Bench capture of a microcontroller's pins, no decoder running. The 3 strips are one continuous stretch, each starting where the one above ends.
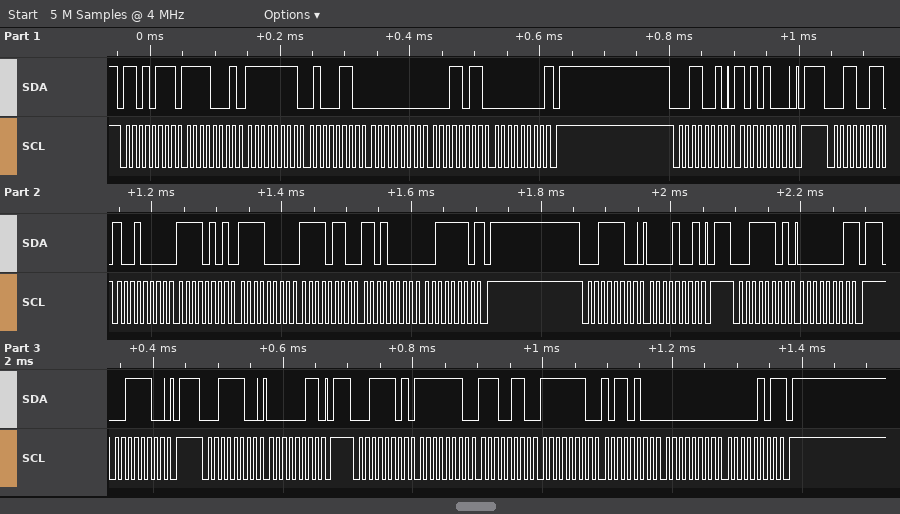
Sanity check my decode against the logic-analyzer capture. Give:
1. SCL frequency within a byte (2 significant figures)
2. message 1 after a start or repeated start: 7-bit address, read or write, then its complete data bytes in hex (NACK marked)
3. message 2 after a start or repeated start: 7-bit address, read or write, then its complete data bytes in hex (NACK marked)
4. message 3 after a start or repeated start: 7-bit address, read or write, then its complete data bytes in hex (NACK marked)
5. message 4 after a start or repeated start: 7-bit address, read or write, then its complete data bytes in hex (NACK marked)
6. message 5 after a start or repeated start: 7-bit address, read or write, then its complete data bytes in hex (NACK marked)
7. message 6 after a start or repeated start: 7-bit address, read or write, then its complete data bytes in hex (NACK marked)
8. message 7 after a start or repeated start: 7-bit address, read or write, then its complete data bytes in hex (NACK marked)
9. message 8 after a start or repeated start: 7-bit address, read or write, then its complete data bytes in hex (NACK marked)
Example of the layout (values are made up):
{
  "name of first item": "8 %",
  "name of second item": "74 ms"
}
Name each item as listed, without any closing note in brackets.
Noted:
{
  "SCL frequency within a byte": "100 kHz",
  "message 1 after a start or repeated start: 7-bit address, read or write, then its complete data bytes in hex": "0x6B read: F1 FF 46 00 1B 00 NACK",
  "message 2 after a start or repeated start: 7-bit address, read or write, then its complete data bytes in hex": "0x19 write: A8",
  "message 3 after a start or repeated start: 7-bit address, read or write, then its complete data bytes in hex": "0x19 read: 90 F5 F0 F6 D0 3E NACK",
  "message 4 after a start or repeated start: 7-bit address, read or write, then its complete data bytes in hex": "0x1E write: 09",
  "message 5 after a start or repeated start: 7-bit address, read or write, then its complete data bytes in hex": "0x1E read: 01 NACK",
  "message 6 after a start or repeated start: 7-bit address, read or write, then its complete data bytes in hex": "0x1E write",
  "message 7 after a start or repeated start: 7-bit address, read or write, then its complete data bytes in hex": "0x1E write: 03",
  "message 8 after a start or repeated start: 7-bit address, read or write, then its complete data bytes in hex": "0x1E read: FE E6 FE B4 00 05 NACK"
}
